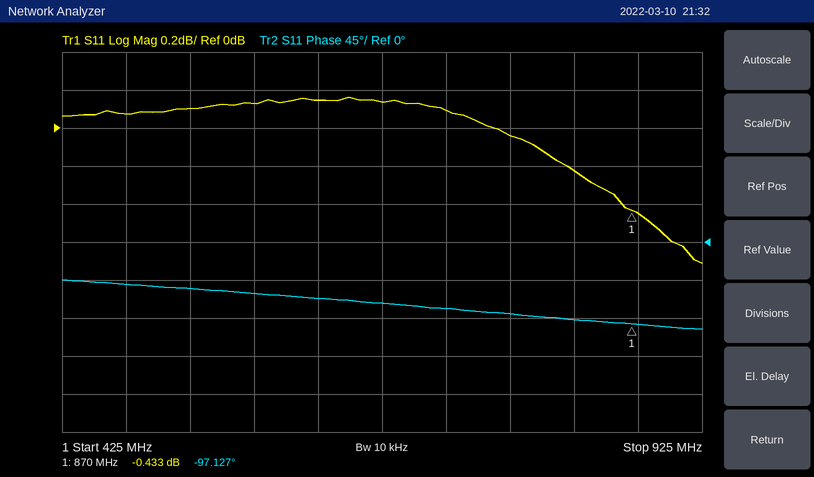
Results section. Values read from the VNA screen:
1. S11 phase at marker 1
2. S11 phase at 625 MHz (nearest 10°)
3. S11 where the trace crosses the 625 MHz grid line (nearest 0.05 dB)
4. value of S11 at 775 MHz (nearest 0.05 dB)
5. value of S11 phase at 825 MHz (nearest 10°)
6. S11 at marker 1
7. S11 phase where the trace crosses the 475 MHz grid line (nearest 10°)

-97.127°
-70°
0.15 dB
-0.05 dB
-90°
-0.433 dB
-50°
